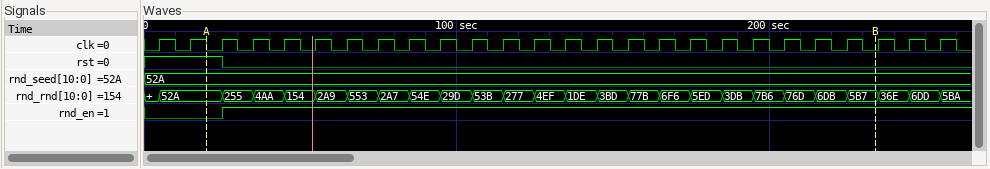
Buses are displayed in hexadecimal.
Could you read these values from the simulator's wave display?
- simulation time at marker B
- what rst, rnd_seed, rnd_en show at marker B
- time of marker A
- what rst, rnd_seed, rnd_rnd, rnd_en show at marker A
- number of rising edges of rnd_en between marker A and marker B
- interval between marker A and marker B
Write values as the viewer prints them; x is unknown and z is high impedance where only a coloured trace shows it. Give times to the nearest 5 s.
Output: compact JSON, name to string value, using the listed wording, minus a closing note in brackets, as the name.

{"simulation time at marker B": "235 s", "what rst, rnd_seed, rnd_en show at marker B": "rst=0, rnd_seed=52A, rnd_en=1", "time of marker A": "20 s", "what rst, rnd_seed, rnd_rnd, rnd_en show at marker A": "rst=1, rnd_seed=52A, rnd_rnd=52A, rnd_en=0", "number of rising edges of rnd_en between marker A and marker B": "1", "interval between marker A and marker B": "215 s"}
